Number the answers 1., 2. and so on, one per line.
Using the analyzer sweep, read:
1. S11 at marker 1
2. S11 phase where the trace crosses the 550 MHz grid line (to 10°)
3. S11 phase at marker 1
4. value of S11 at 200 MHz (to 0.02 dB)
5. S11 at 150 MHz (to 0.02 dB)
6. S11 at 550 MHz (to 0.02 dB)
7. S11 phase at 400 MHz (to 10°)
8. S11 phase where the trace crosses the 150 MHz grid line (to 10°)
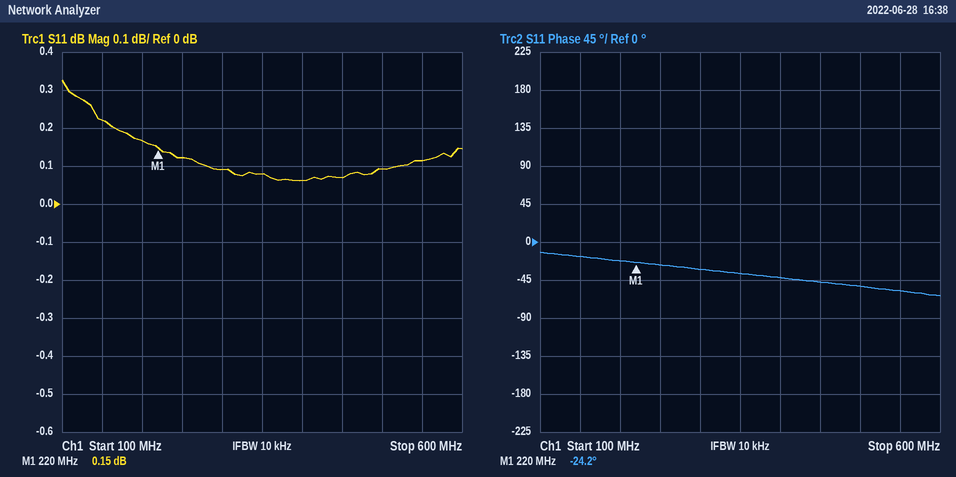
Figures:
1. 0.15 dB
2. -60°
3. -24.2°
4. 0.16 dB
5. 0.22 dB
6. 0.12 dB
7. -40°
8. -20°
